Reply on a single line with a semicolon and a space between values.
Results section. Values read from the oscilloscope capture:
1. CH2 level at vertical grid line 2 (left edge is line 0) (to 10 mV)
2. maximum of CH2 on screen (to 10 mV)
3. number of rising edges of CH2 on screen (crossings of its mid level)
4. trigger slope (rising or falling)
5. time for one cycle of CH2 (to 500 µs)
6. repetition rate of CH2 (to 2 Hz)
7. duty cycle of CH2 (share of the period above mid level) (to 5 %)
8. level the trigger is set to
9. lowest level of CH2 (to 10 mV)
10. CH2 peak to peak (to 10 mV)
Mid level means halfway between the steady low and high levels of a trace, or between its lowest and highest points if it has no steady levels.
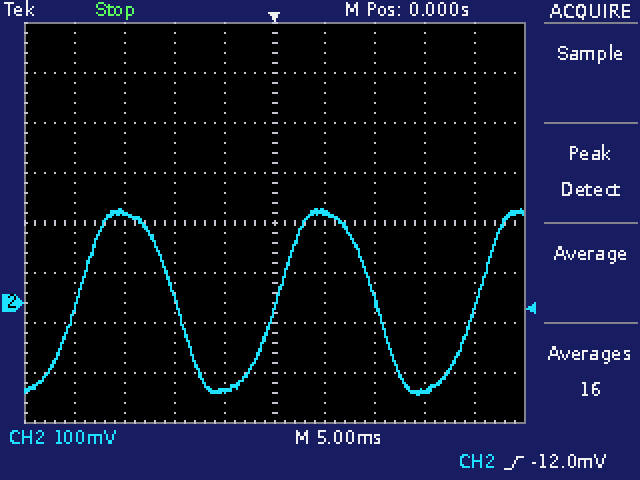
180 mV; 190 mV; 3; rising; 20.0 ms; 50 Hz; 50 %; -12.0 mV; -180 mV; 370 mV
